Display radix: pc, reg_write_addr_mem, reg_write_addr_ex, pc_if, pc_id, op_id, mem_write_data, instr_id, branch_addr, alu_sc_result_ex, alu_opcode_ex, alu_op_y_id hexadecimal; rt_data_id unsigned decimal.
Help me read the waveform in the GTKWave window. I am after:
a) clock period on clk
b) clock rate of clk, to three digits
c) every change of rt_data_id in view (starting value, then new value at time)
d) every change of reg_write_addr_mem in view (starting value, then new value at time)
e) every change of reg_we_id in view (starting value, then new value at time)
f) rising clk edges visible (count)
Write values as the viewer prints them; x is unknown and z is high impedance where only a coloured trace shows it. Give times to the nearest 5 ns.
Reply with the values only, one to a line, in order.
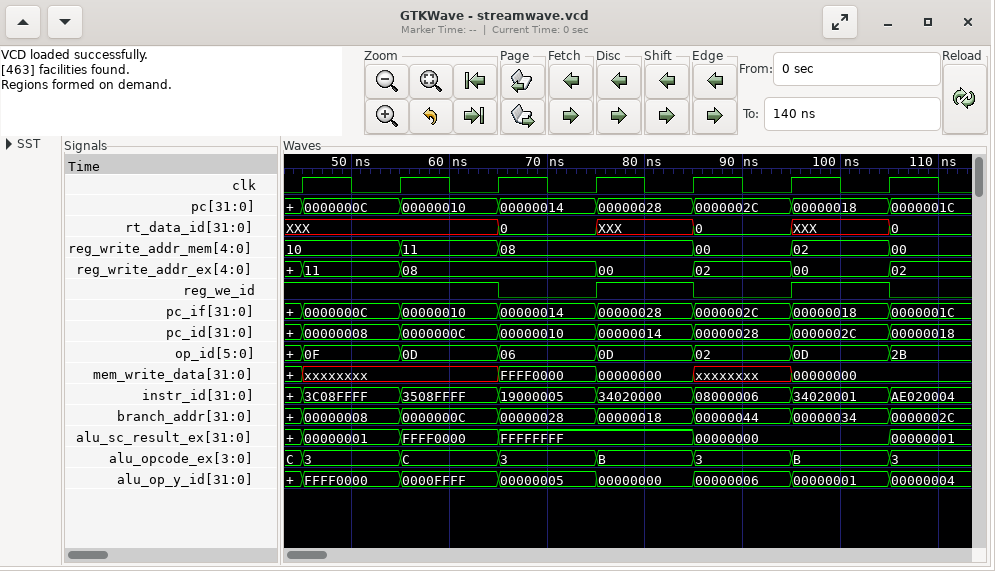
10 ns
100 MHz
XXX, 0 at 65 ns, XXX at 75 ns, 0 at 85 ns, XXX at 95 ns, 0 at 105 ns
10, 11 at 55 ns, 08 at 65 ns, 00 at 85 ns, 02 at 95 ns, 00 at 105 ns
1, 0 at 65 ns, 1 at 75 ns, 0 at 85 ns, 1 at 95 ns, 0 at 105 ns
7
